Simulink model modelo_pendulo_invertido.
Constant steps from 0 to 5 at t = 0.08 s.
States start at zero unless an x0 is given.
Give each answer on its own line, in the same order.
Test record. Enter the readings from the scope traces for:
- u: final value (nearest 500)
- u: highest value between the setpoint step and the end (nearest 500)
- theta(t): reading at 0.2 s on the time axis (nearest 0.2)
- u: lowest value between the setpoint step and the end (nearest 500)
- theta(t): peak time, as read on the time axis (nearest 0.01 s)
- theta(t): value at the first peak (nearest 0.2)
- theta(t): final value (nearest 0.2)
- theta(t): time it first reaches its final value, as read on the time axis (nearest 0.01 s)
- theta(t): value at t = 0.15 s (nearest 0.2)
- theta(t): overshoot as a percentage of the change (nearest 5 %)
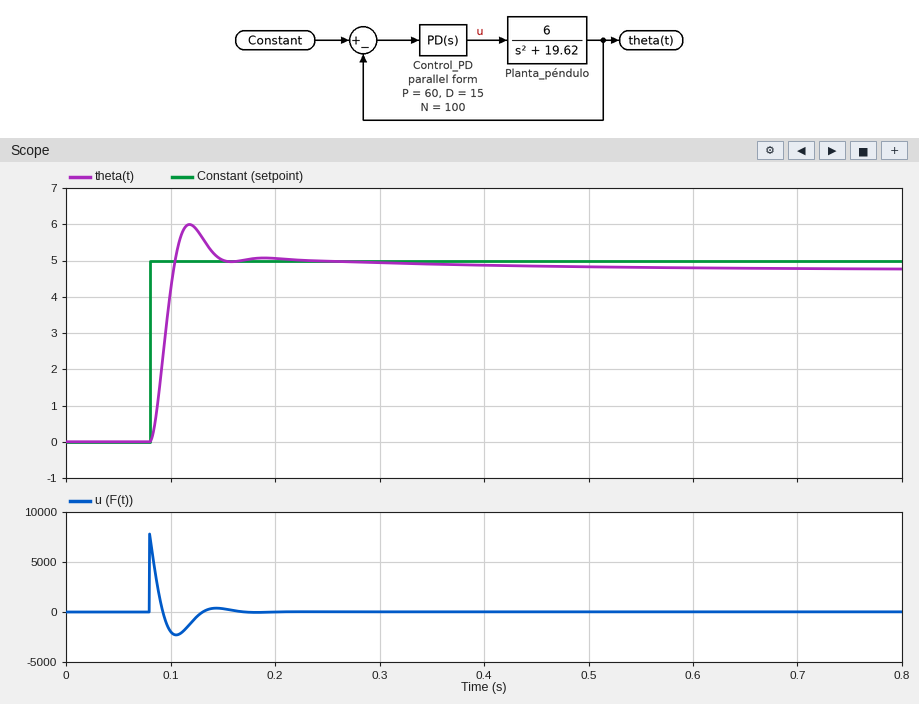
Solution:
0
8000
5.0
-2500
0.12 s
6.0
4.8
0.10 s
5.0
25 %
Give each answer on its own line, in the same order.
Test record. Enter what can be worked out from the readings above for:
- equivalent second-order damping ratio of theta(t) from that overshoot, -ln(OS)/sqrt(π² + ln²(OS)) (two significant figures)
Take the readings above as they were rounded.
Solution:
0.40
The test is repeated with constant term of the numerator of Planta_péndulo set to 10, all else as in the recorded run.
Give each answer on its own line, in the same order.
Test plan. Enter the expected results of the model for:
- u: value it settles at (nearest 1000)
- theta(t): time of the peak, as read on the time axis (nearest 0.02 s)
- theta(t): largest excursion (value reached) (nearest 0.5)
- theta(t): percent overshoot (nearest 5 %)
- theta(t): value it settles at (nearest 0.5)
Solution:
0
0.10 s
6.5
35 %
5.0
